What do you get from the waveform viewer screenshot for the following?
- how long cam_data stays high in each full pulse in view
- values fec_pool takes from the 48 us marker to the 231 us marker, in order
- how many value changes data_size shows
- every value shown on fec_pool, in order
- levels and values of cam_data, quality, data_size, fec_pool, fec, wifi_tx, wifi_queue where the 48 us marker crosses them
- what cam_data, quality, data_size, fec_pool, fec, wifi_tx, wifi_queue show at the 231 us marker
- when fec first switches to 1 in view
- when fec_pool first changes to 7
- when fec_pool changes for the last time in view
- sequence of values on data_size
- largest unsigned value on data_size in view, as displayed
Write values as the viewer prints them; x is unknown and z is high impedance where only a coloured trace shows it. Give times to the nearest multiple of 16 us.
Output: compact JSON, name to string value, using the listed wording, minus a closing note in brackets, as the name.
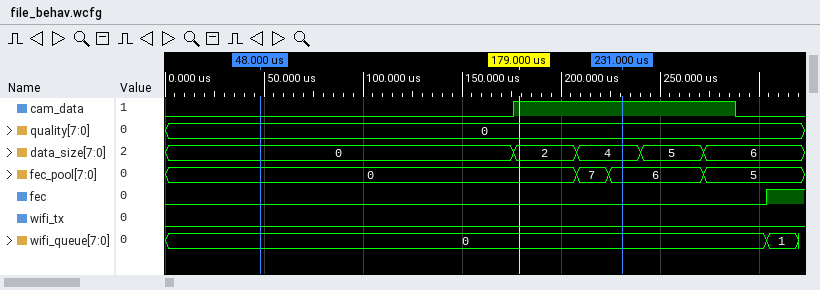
{"how long cam_data stays high in each full pulse in view": "112 us", "values fec_pool takes from the 48 us marker to the 231 us marker, in order": "0, 7, 6", "how many value changes data_size shows": "4", "every value shown on fec_pool, in order": "0, 7, 6, 5", "levels and values of cam_data, quality, data_size, fec_pool, fec, wifi_tx, wifi_queue where the 48 us marker crosses them": "cam_data=0, quality=0, data_size=0, fec_pool=0, fec=0, wifi_tx=0, wifi_queue=0", "what cam_data, quality, data_size, fec_pool, fec, wifi_tx, wifi_queue show at the 231 us marker": "cam_data=1, quality=0, data_size=4, fec_pool=6, fec=0, wifi_tx=0, wifi_queue=0", "when fec first switches to 1 in view": "304 us", "when fec_pool first changes to 7": "208 us", "when fec_pool changes for the last time in view": "272 us", "sequence of values on data_size": "0, 2, 4, 5, 6", "largest unsigned value on data_size in view, as displayed": "6"}
